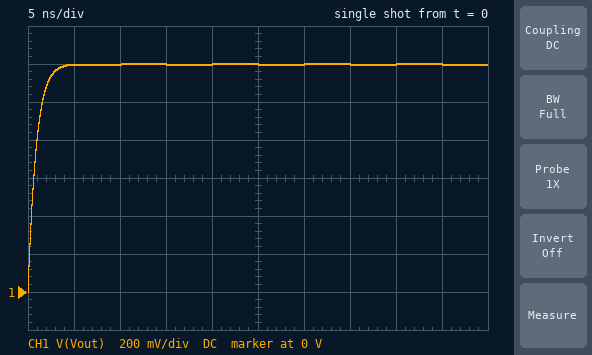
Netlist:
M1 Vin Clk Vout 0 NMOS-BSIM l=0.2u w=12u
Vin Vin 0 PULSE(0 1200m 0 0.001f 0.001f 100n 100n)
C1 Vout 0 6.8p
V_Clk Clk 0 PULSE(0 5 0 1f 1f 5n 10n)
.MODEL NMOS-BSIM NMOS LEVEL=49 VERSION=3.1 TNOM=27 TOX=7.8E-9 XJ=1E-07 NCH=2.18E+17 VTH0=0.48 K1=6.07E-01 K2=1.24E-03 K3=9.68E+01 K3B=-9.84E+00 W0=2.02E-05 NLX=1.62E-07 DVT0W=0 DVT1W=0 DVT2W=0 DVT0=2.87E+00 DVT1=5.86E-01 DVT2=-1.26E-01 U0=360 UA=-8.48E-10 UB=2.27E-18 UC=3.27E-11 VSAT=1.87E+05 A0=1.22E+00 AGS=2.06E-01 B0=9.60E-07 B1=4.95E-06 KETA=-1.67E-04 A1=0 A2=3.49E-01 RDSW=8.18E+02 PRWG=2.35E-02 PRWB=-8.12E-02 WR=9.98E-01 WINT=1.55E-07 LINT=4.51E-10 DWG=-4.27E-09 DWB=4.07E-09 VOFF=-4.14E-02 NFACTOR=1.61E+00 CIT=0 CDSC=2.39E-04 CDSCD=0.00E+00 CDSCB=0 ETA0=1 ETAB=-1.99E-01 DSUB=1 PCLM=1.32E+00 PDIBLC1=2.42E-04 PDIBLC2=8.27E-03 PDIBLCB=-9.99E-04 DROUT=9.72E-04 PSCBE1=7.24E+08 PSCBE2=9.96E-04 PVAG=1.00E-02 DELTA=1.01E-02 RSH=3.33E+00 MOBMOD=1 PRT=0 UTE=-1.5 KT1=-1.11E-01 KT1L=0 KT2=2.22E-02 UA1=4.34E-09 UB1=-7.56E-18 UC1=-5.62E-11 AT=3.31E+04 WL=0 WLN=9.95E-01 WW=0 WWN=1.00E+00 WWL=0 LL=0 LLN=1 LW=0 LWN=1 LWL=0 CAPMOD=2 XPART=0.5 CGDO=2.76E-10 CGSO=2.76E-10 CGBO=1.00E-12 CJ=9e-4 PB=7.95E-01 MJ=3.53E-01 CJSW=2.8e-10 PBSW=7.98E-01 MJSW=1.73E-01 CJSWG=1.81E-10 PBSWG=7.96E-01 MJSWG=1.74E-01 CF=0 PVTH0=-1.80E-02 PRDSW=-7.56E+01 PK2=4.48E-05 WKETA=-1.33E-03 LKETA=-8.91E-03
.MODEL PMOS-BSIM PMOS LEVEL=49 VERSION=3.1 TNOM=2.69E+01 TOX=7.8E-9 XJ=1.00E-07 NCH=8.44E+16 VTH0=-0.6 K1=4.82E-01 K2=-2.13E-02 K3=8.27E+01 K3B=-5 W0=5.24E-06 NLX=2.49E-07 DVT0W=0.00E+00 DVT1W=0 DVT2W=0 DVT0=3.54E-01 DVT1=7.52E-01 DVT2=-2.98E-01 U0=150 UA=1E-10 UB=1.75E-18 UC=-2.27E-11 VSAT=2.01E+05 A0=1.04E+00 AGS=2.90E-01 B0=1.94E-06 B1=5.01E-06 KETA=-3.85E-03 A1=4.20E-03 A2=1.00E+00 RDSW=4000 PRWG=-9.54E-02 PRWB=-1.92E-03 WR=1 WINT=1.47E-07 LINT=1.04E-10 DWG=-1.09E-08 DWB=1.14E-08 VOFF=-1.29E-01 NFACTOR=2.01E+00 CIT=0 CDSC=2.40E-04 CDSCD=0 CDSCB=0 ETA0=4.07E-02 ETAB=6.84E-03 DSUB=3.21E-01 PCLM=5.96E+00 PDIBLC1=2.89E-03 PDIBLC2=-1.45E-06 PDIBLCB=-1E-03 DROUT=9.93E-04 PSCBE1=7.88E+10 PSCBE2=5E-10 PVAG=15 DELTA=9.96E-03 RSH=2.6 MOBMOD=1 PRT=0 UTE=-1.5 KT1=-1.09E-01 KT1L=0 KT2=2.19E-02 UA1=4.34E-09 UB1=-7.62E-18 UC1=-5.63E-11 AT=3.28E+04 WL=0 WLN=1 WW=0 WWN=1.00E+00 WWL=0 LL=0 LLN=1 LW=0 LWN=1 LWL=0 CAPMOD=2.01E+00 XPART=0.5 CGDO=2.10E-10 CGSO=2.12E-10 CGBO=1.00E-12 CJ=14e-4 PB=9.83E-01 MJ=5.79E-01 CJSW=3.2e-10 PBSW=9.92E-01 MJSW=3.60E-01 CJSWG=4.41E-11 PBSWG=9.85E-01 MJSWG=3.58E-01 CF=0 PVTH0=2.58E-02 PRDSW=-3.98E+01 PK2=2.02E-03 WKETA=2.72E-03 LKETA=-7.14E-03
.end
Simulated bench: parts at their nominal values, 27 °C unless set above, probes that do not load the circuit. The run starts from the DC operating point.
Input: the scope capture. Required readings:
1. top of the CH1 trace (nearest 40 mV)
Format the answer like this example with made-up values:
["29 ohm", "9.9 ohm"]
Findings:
["1.20 V"]
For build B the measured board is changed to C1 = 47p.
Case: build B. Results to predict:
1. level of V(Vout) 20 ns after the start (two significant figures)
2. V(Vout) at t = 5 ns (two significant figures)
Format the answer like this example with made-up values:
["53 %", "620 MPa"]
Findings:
["970 mV", "660 mV"]
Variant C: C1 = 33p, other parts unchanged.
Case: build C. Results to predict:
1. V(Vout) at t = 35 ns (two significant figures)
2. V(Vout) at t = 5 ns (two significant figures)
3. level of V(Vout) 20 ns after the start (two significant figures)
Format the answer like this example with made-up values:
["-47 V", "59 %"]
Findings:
["1.2 V", "820 mV", "1.1 V"]
